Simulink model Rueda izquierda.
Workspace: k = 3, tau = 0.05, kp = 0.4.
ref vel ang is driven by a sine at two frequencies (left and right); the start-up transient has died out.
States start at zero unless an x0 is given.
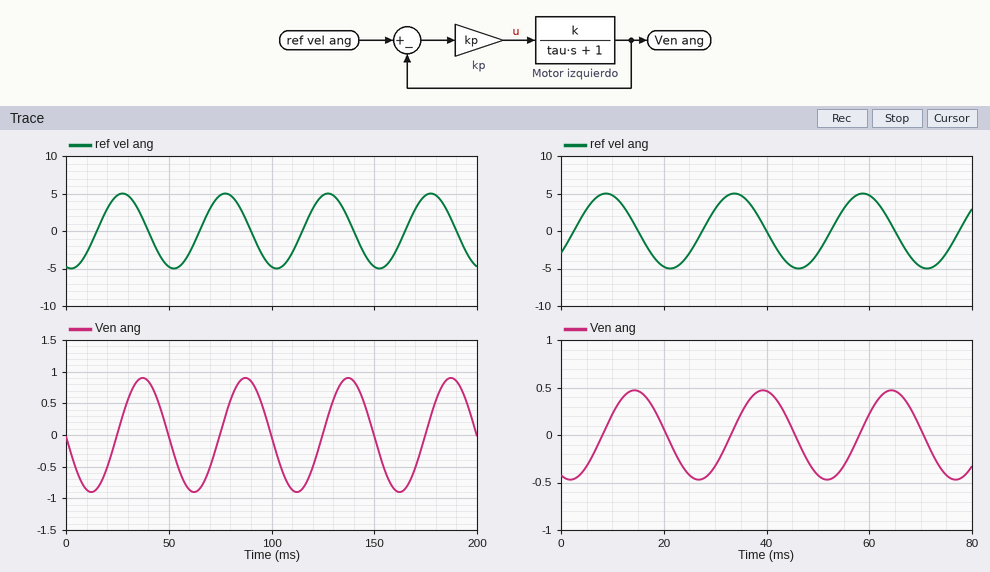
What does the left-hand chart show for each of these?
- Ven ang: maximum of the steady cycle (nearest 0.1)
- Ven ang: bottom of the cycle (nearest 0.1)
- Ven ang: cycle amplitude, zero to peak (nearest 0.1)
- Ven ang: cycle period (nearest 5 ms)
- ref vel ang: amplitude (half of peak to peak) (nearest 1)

0.9
-0.9
0.9
50 ms
5
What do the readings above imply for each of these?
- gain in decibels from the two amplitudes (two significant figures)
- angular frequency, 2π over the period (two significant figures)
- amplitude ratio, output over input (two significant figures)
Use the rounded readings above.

-15 dB
0.13 rad/ms
0.18
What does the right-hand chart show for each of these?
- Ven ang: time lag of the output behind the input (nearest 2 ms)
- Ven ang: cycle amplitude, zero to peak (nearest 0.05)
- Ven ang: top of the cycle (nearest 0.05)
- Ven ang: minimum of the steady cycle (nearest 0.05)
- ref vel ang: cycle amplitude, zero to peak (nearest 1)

6 ms
0.45
0.45
-0.45
5
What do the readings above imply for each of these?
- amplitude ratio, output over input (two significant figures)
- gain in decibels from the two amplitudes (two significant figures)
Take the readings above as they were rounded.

0.090
-21 dB
